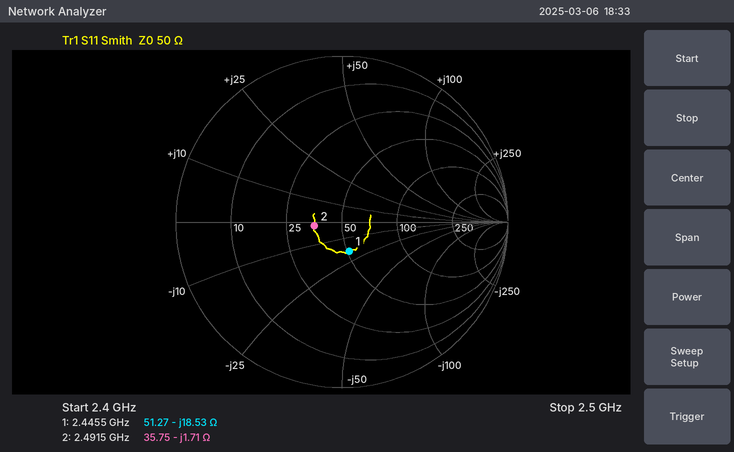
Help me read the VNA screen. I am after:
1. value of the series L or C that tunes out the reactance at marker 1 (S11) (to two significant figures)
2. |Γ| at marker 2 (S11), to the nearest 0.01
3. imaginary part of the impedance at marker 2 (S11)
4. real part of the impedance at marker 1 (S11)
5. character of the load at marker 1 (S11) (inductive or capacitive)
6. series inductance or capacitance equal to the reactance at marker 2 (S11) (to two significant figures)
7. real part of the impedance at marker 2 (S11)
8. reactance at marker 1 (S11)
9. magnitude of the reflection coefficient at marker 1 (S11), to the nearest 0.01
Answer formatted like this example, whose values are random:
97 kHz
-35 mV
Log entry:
1.2 nH
0.17
-1.71 Ω
51.27 Ω
capacitive
37 pF
35.75 Ω
-18.53 Ω
0.18
